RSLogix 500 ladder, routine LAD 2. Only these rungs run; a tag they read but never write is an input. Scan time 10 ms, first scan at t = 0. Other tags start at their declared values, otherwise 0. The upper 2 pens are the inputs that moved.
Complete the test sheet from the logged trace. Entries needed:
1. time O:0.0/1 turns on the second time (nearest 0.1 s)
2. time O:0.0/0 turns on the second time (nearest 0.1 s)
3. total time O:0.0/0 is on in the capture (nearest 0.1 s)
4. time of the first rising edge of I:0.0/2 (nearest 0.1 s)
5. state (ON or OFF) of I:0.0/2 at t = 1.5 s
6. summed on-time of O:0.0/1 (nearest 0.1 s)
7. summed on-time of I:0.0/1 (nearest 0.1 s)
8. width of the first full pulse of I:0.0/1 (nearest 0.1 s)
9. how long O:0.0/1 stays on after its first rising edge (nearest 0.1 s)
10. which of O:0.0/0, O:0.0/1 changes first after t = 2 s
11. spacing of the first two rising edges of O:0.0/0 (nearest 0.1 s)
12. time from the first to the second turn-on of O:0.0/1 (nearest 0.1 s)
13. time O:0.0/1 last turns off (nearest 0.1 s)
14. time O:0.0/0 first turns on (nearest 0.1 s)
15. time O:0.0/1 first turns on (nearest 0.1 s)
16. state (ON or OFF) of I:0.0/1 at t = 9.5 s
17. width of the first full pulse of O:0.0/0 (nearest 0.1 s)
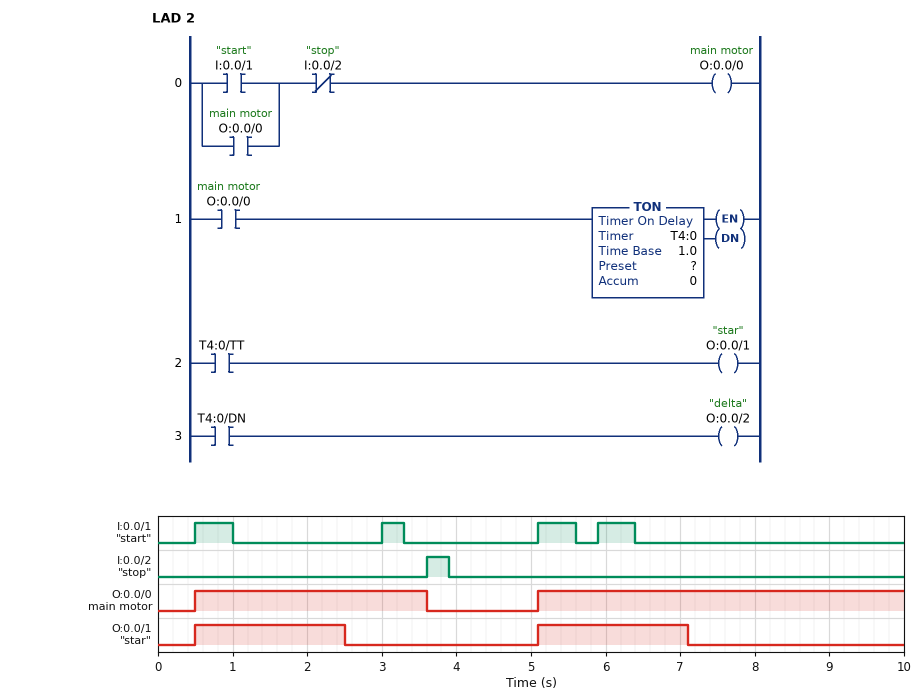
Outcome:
5.1 s
5.1 s
8.0 s
3.6 s
OFF
4.0 s
1.8 s
0.5 s
2.0 s
O:0.0/1
4.6 s
4.6 s
7.1 s
0.5 s
0.5 s
OFF
3.1 s
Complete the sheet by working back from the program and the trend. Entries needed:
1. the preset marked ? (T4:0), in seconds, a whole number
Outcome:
2 s
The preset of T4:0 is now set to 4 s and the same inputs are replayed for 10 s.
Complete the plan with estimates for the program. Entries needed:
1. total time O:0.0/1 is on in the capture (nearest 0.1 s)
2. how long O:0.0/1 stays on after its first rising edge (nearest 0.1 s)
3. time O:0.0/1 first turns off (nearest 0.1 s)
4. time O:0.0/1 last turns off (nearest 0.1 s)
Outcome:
7.1 s
3.1 s
3.6 s
9.1 s
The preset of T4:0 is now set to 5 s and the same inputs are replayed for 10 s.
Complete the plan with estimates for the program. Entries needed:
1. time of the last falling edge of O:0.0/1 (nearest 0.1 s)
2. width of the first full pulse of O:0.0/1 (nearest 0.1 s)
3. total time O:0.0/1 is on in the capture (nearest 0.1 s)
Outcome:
3.6 s
3.1 s
8.0 s
